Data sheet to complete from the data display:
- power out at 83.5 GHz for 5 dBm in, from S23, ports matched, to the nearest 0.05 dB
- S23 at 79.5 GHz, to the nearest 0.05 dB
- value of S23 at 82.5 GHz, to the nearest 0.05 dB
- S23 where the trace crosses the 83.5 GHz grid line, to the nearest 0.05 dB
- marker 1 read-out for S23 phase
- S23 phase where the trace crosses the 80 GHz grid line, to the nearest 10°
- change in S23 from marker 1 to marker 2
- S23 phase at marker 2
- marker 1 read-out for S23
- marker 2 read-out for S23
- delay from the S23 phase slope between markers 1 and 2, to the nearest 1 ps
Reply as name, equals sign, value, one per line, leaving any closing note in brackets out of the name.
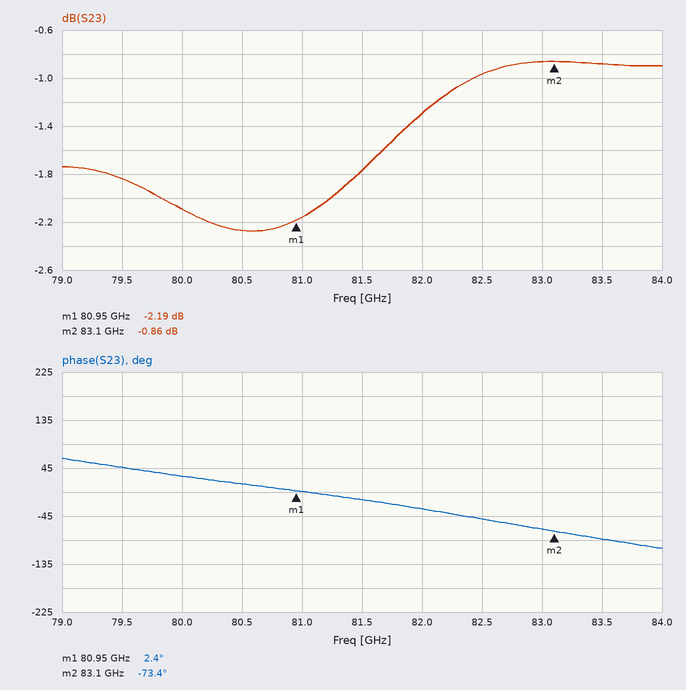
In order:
power out at 83.5 GHz for 5 dBm in, from S23, ports matched, to the nearest 0.05 dB = 4.10 dBm
S23 at 79.5 GHz, to the nearest 0.05 dB = -1.85 dB
value of S23 at 82.5 GHz, to the nearest 0.05 dB = -0.95 dB
S23 where the trace crosses the 83.5 GHz grid line, to the nearest 0.05 dB = -0.90 dB
marker 1 read-out for S23 phase = 2.4°
S23 phase where the trace crosses the 80 GHz grid line, to the nearest 10° = 30°
change in S23 from marker 1 to marker 2 = 1.33 dB
S23 phase at marker 2 = -73.4°
marker 1 read-out for S23 = -2.19 dB
marker 2 read-out for S23 = -0.86 dB
delay from the S23 phase slope between markers 1 and 2, to the nearest 1 ps = 98 ps
